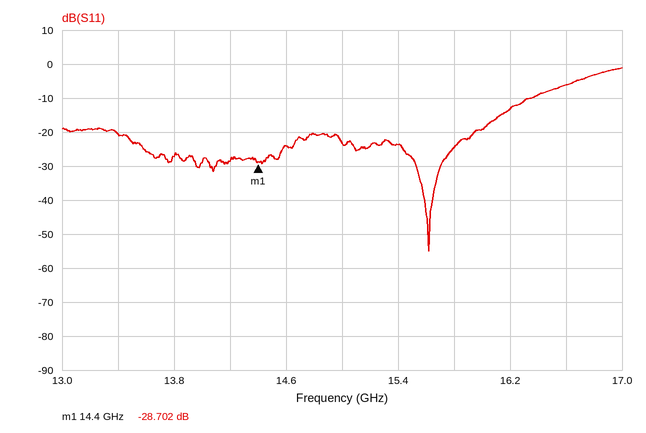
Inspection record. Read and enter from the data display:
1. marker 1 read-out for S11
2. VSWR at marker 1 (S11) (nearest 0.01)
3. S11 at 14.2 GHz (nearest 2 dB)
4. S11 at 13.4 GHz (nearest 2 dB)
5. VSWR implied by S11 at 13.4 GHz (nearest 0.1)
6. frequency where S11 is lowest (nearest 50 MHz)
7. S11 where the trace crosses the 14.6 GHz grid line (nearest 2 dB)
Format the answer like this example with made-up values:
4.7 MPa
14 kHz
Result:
-28.702 dB
1.08
-28 dB
-20 dB
1.2
15.60 GHz
-24 dB
